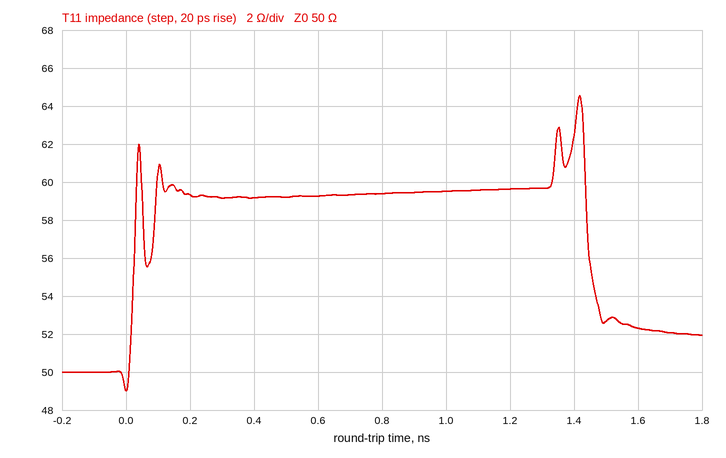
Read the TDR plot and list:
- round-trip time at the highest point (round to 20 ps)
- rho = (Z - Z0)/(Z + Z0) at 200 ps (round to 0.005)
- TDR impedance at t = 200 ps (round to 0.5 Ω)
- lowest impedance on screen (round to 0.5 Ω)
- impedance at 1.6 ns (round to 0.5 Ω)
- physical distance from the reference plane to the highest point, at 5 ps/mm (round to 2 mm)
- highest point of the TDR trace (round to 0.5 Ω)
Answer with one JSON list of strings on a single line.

["1.42 ns", "+0.085", "59.5 Ω", "49.0 Ω", "52.5 Ω", "142 mm", "64.5 Ω"]
